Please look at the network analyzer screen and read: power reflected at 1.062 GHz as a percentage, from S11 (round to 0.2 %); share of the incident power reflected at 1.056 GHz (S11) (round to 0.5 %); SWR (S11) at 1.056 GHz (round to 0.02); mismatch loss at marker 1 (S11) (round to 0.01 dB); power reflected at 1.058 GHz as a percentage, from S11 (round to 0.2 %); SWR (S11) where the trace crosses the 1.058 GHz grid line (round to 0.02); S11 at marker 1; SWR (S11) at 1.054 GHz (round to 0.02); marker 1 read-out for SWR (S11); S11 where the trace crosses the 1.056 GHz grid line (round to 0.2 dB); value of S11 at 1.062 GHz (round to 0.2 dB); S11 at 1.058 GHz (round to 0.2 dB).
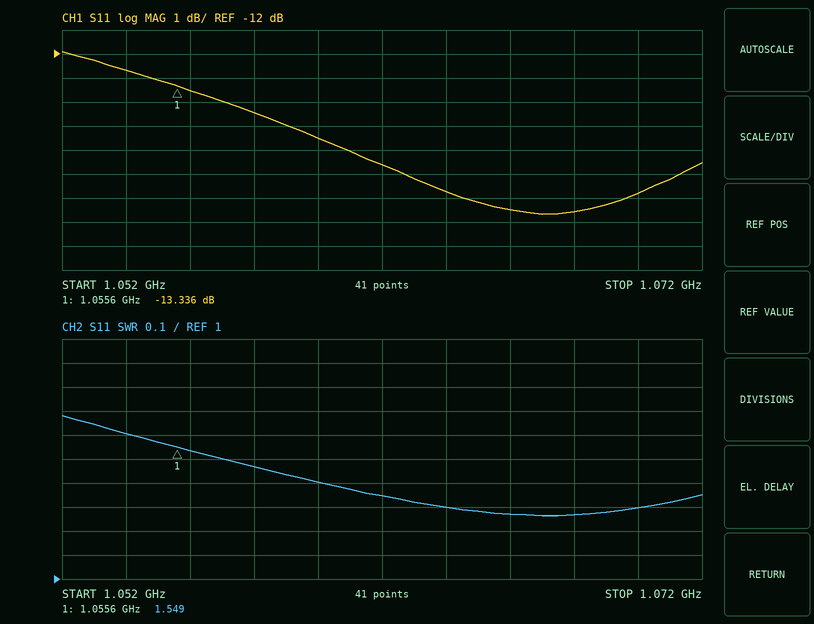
2.2 %
4.5 %
1.54
0.21 dB
3.6 %
1.46
-13.336 dB
1.60
1.549
-13.6 dB
-16.6 dB
-14.4 dB
